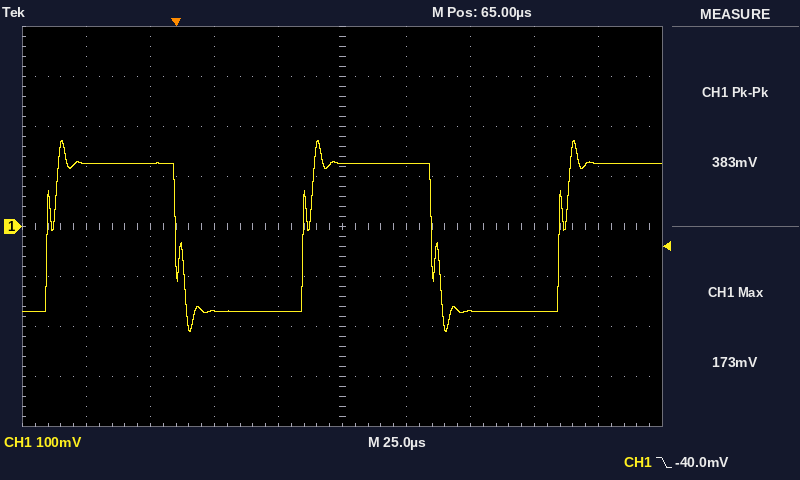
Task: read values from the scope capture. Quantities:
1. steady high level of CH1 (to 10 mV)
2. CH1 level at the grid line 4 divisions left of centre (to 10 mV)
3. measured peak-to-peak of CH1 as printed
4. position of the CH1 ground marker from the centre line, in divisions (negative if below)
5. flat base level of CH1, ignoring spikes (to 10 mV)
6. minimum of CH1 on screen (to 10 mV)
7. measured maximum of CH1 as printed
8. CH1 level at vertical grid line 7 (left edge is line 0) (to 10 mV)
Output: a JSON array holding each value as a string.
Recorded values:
["130 mV", "130 mV", "383 mV", "0.0 div", "-170 mV", "-210 mV", "173 mV", "-170 mV"]
